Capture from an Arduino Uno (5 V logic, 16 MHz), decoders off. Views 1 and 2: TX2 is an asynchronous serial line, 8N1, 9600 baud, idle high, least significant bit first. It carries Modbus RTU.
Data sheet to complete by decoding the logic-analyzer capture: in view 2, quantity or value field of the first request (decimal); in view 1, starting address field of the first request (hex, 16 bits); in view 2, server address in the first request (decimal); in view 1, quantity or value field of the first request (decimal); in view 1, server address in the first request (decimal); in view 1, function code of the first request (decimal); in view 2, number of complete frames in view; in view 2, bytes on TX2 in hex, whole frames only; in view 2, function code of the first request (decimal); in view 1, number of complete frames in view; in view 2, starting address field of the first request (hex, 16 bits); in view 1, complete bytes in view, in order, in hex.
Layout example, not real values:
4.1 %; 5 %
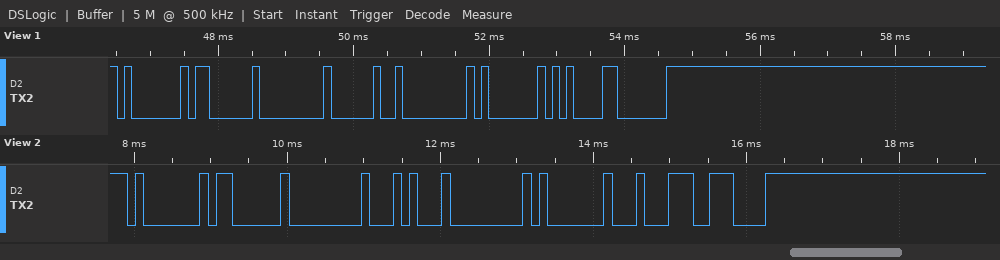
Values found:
1; 0x0020; 1; 1; 1; 3; 8; 01 03 00 14 00 01 C4 0E; 3; 8; 0x0014; 0x01 0x03 0x00 0x20 0x00 0x01 0x85 0xC0
